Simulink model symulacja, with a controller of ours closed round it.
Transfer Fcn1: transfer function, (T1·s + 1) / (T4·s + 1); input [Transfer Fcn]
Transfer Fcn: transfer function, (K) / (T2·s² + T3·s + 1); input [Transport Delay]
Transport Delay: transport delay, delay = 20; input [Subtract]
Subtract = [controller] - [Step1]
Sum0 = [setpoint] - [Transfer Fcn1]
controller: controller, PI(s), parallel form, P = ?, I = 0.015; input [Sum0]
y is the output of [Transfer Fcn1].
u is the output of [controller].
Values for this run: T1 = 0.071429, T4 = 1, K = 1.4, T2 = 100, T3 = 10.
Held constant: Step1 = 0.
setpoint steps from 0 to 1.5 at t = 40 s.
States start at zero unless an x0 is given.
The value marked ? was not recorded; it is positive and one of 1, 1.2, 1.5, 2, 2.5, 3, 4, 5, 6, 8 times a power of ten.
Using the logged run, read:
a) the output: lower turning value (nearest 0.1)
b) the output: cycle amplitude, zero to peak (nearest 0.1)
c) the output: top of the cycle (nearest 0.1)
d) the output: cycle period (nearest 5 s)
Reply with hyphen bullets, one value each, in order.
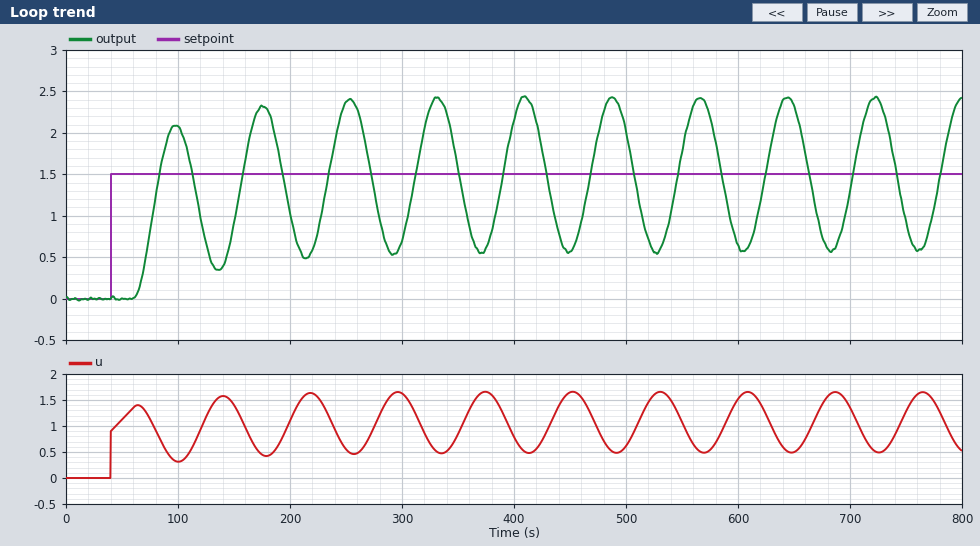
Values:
- 0.6
- 0.9
- 2.4
- 80 s
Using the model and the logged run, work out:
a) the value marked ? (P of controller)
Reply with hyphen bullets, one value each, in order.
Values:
- 0.6
